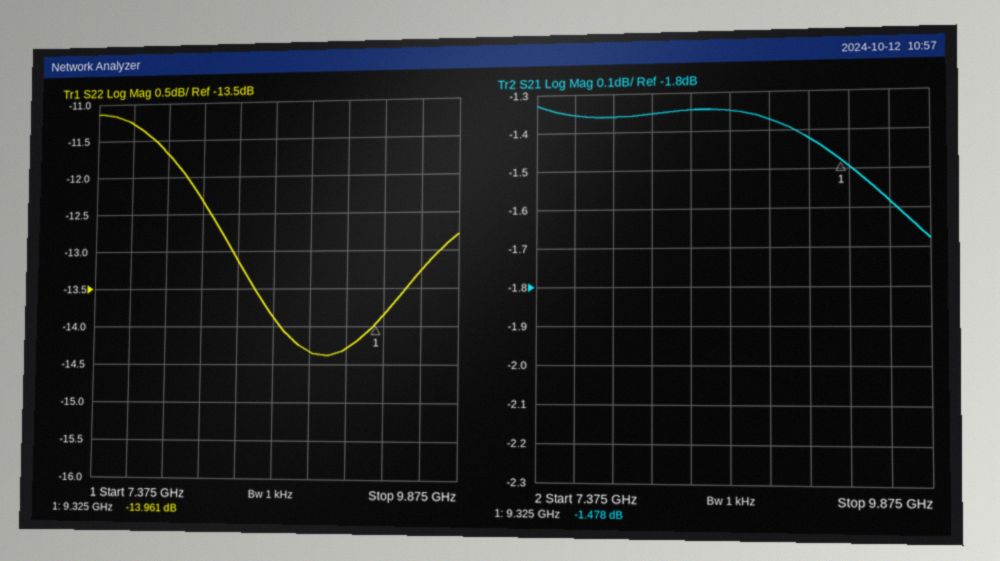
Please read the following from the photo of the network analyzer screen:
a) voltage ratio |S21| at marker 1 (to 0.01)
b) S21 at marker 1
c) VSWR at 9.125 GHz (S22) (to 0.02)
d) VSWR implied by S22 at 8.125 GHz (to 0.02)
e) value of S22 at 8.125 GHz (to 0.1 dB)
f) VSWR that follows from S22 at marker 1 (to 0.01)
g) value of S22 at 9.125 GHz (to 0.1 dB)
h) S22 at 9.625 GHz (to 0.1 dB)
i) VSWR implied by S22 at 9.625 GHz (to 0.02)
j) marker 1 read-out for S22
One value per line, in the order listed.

0.84
-1.478 dB
1.48
1.64
-12.3 dB
1.50
-14.3 dB
-13.3 dB
1.56
-13.961 dB
